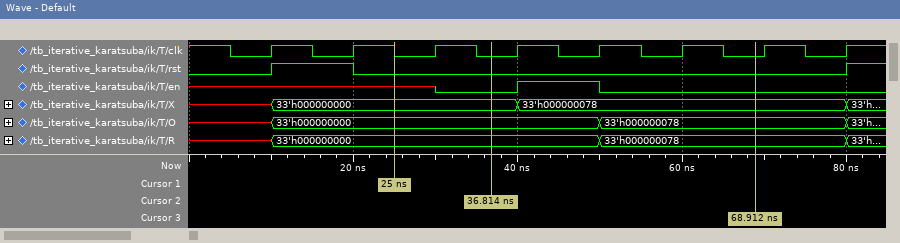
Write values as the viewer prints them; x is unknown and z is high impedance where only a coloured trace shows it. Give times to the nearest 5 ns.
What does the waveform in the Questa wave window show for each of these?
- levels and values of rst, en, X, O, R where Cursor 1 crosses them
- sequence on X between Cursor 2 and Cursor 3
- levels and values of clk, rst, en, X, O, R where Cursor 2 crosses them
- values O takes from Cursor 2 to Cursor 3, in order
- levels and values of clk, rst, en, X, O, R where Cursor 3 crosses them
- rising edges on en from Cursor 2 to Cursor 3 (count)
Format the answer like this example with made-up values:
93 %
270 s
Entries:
rst=0, en=x, X=33'h000000000, O=33'h000000000, R=33'h000000000
33'h000000000, 33'h000000078
clk=0, rst=0, en=0, X=33'h000000000, O=33'h000000000, R=33'h000000000
33'h000000000, 33'h000000078
clk=0, rst=0, en=0, X=33'h000000078, O=33'h000000078, R=33'h000000078
1
